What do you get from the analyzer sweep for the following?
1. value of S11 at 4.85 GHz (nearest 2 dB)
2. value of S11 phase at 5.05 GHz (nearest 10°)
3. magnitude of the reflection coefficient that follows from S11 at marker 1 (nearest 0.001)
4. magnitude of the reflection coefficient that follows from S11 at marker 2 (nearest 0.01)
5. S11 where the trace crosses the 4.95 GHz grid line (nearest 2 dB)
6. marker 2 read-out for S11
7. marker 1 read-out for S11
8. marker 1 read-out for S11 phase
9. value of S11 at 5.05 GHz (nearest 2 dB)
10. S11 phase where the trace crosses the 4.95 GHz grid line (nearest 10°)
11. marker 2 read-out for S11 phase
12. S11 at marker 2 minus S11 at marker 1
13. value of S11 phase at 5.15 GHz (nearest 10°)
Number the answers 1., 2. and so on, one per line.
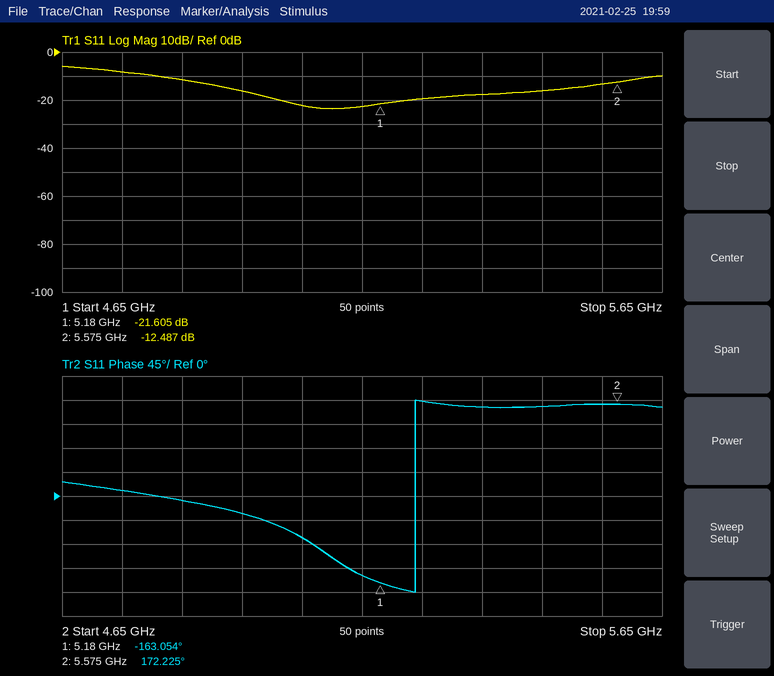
1. -12 dB
2. -80°
3. 0.083
4. 0.24
5. -16 dB
6. -12.487 dB
7. -21.605 dB
8. -163.054°
9. -22 dB
10. -30°
11. 172.225°
12. 9.118 dB
13. -150°
